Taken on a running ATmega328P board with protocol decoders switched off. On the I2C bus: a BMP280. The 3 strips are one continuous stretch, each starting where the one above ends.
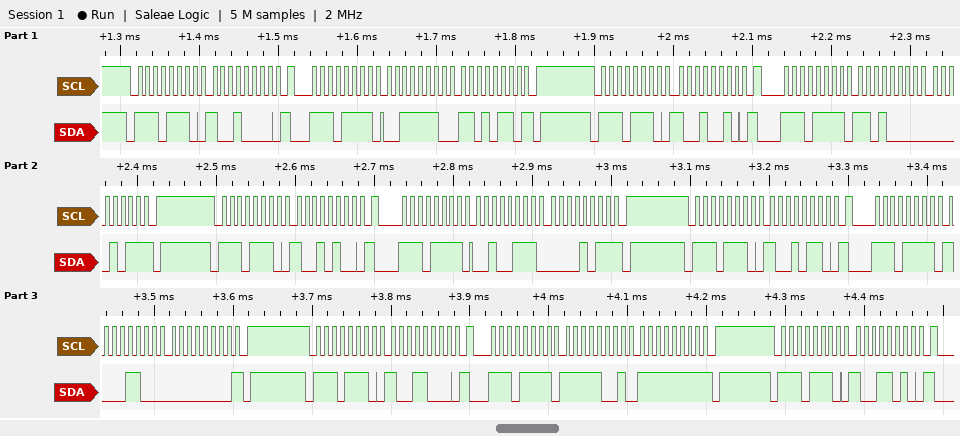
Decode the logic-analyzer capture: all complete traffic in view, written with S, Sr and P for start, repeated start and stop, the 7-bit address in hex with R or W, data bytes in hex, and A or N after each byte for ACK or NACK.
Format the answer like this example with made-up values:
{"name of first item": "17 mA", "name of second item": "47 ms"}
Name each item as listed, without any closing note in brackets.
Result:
{"all complete traffic in view, written with S, Sr and P for start, repeated start and stop, the 7-bit address in hex with R or W, data bytes in hex, and A or N after each byte for ACK or NACK": "S 77W A 90 A Sr 77R A 3E A D6 N P S 77W A 92 A Sr 77R A D0 A 0B N P S 77W A 94 A Sr 77R A 27 A 0B N P S 77W A 96 A Sr 77R A 8C A 00 N P S 77W A 98 A Sr 77R A F9 A FF N P S 77W A 9A A"}
